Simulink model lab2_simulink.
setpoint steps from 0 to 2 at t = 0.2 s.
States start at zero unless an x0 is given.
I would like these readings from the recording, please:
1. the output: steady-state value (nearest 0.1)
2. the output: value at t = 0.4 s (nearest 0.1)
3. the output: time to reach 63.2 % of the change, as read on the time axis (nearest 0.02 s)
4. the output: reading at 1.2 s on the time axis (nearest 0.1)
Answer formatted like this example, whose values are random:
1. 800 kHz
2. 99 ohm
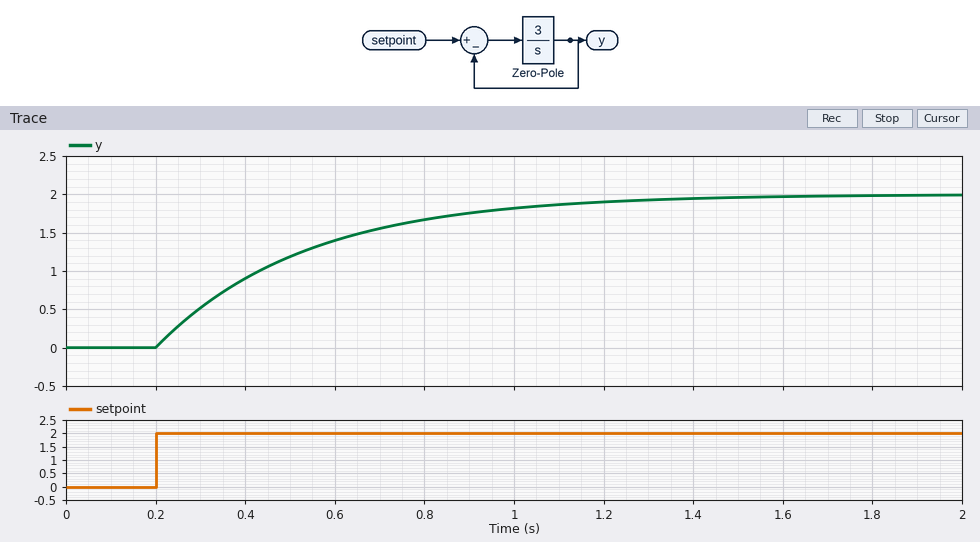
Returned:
1. 2.0
2. 0.9
3. 0.54 s
4. 1.9
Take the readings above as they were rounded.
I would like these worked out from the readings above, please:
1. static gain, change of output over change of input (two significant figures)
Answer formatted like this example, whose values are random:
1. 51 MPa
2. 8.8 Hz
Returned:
1. 1.0
